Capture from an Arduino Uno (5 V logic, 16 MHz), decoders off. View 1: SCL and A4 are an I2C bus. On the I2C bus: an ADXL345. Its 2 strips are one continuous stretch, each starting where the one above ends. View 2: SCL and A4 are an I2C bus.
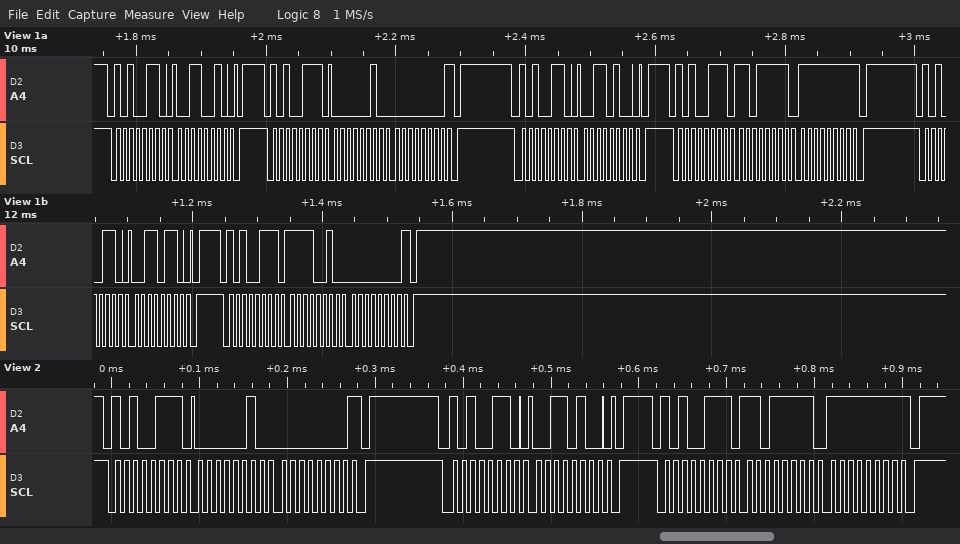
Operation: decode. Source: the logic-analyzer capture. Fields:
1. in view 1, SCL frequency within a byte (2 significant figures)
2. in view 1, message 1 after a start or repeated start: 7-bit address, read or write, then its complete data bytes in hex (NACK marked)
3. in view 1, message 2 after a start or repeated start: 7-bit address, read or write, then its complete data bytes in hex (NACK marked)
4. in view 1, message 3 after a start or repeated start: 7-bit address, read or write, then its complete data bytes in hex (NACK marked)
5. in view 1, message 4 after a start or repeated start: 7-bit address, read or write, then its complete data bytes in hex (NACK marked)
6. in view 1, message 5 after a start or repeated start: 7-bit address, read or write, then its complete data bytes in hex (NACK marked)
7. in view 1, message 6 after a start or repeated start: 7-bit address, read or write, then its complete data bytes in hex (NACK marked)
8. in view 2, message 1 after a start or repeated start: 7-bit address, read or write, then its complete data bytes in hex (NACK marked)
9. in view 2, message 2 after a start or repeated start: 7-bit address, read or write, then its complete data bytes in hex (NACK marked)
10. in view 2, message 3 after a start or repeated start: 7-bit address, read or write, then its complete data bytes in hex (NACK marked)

100 kHz
0x53 write: 32
0x53 read: 02 00 NACK
0x53 write: 34
0x53 read: DF FF NACK
0x53 write: 36
0x53 read: F2 00 NACK
0x53 read: 02 00 NACK
0x53 write: 34
0x53 read: DF FF NACK
